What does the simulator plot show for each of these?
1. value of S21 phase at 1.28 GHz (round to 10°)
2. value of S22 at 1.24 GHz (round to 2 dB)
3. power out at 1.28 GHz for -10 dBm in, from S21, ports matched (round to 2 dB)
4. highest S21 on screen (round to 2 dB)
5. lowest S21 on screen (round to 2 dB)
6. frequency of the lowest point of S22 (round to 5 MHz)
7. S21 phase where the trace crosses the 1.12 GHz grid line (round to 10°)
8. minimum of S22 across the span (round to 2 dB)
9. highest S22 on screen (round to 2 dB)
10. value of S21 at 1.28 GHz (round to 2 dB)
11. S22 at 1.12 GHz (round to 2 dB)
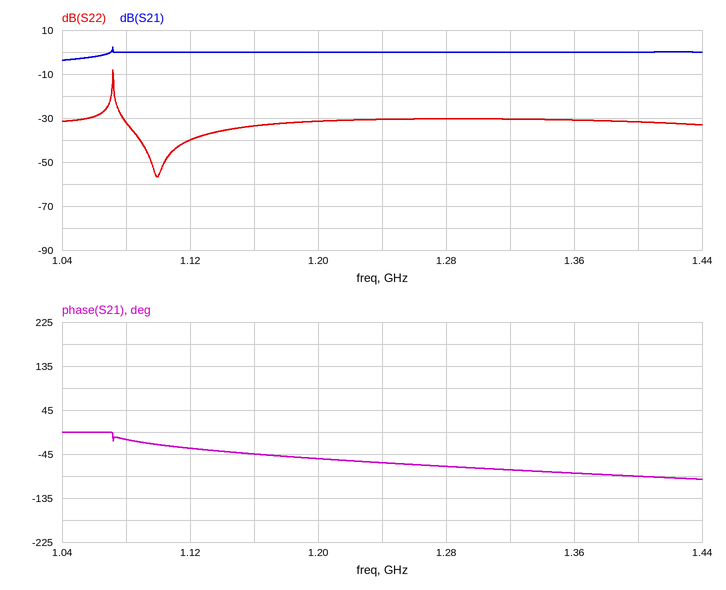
-70°
-30 dB
-10 dBm
2 dB
-4 dB
1.100 GHz
-30°
-56 dB
-8 dB
0 dB
-40 dB
